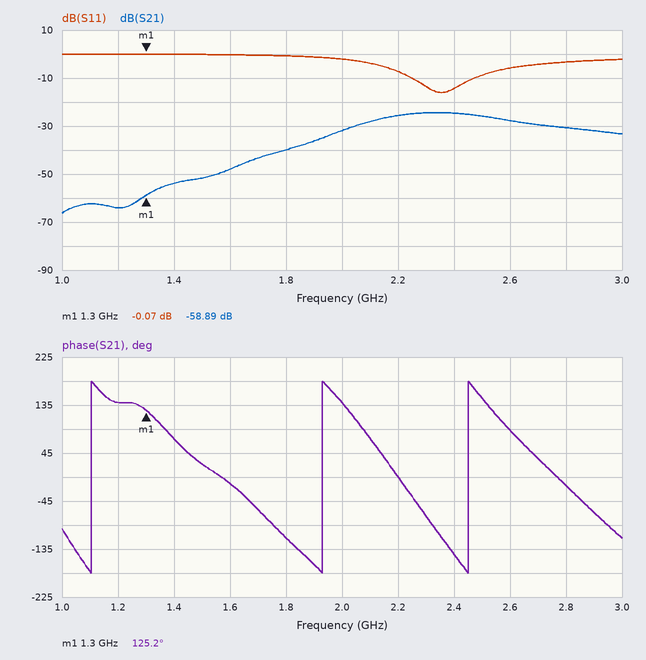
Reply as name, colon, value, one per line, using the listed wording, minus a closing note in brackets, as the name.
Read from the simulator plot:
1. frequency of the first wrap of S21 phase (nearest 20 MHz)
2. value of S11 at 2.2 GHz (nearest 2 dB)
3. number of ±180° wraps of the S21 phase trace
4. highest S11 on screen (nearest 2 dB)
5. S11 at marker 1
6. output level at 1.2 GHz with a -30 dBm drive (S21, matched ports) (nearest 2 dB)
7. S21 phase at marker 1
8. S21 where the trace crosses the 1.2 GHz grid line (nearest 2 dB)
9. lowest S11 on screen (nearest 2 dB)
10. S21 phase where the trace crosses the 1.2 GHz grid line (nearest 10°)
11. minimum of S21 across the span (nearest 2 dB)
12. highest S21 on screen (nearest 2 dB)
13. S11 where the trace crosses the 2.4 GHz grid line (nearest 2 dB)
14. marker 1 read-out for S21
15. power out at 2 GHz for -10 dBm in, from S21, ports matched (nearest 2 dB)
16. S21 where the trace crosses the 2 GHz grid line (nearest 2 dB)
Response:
frequency of the first wrap of S21 phase: 1.10 GHz
value of S11 at 2.2 GHz: -8 dB
number of ±180° wraps of the S21 phase trace: 3
highest S11 on screen: 0 dB
S11 at marker 1: -0.07 dB
output level at 1.2 GHz with a -30 dBm drive (S21, matched ports): -94 dBm
S21 phase at marker 1: 125.2°
S21 where the trace crosses the 1.2 GHz grid line: -64 dB
lowest S11 on screen: -16 dB
S21 phase where the trace crosses the 1.2 GHz grid line: 140°
minimum of S21 across the span: -66 dB
highest S21 on screen: -24 dB
S11 where the trace crosses the 2.4 GHz grid line: -14 dB
marker 1 read-out for S21: -58.89 dB
power out at 2 GHz for -10 dBm in, from S21, ports matched: -42 dBm
S21 where the trace crosses the 2 GHz grid line: -32 dB
